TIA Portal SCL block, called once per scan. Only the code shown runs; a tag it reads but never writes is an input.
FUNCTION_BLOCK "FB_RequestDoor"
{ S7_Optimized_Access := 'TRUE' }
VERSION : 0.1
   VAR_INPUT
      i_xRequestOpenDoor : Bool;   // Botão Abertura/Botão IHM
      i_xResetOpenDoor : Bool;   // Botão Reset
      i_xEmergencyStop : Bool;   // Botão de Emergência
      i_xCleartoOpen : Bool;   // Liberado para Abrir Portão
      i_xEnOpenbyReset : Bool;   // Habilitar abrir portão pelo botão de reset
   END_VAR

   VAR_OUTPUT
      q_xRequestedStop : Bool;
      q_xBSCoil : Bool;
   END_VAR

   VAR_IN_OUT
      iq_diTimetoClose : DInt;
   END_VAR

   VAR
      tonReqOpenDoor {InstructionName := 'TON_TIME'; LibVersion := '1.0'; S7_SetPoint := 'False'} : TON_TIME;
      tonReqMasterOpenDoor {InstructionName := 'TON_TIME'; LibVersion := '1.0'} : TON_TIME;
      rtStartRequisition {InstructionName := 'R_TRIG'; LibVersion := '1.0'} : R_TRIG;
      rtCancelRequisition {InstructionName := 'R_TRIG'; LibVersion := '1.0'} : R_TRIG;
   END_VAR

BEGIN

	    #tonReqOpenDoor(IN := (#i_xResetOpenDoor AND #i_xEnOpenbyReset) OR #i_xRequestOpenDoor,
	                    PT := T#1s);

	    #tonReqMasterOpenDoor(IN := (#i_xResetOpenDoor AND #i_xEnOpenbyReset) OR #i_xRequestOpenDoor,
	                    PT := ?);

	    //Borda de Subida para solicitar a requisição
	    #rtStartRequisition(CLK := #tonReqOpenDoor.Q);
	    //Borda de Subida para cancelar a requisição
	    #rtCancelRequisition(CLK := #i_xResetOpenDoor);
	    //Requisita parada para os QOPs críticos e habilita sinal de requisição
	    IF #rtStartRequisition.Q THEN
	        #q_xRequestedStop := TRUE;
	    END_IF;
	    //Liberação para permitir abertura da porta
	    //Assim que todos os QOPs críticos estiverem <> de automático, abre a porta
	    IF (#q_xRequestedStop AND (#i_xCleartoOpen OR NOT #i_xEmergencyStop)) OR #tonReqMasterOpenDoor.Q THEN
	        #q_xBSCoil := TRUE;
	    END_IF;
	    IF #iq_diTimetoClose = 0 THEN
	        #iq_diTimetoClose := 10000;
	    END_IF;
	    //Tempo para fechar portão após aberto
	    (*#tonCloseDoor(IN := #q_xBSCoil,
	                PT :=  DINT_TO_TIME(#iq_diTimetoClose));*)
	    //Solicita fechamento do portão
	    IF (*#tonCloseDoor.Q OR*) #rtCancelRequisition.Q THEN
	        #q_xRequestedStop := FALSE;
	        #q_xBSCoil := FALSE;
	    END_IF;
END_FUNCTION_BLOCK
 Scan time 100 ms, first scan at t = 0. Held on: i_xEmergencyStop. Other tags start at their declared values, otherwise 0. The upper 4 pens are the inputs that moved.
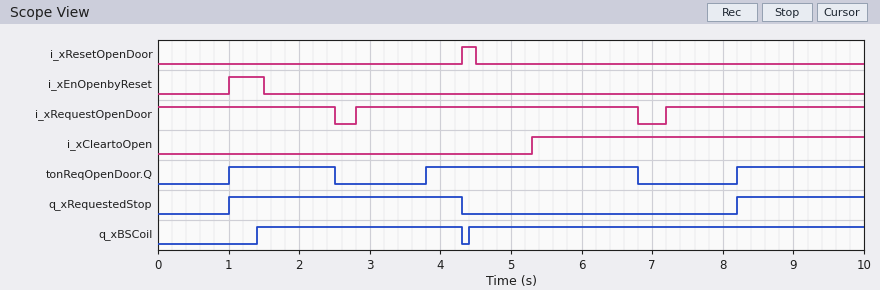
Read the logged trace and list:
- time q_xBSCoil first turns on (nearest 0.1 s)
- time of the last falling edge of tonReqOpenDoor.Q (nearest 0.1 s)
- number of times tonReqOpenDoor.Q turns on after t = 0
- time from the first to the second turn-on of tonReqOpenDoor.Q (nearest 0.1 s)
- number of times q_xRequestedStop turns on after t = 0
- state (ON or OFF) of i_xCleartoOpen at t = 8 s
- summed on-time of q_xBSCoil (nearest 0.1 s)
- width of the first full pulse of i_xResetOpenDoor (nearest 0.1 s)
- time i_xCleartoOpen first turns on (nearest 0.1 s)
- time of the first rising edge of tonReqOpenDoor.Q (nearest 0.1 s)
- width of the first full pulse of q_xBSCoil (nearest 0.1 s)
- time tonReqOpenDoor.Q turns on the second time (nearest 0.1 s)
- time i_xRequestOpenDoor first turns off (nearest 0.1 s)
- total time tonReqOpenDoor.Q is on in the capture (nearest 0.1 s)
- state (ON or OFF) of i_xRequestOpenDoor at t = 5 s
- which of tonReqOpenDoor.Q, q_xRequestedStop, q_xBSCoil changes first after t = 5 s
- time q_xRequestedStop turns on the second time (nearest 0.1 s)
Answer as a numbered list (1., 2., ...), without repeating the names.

1. 1.4 s
2. 6.8 s
3. 3
4. 2.8 s
5. 2
6. ON
7. 8.5 s
8. 0.2 s
9. 5.3 s
10. 1.0 s
11. 2.9 s
12. 3.8 s
13. 2.5 s
14. 6.3 s
15. ON
16. tonReqOpenDoor.Q
17. 8.2 s
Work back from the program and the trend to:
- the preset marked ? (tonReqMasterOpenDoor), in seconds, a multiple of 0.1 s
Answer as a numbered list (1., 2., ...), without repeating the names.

1. 1.4 s
